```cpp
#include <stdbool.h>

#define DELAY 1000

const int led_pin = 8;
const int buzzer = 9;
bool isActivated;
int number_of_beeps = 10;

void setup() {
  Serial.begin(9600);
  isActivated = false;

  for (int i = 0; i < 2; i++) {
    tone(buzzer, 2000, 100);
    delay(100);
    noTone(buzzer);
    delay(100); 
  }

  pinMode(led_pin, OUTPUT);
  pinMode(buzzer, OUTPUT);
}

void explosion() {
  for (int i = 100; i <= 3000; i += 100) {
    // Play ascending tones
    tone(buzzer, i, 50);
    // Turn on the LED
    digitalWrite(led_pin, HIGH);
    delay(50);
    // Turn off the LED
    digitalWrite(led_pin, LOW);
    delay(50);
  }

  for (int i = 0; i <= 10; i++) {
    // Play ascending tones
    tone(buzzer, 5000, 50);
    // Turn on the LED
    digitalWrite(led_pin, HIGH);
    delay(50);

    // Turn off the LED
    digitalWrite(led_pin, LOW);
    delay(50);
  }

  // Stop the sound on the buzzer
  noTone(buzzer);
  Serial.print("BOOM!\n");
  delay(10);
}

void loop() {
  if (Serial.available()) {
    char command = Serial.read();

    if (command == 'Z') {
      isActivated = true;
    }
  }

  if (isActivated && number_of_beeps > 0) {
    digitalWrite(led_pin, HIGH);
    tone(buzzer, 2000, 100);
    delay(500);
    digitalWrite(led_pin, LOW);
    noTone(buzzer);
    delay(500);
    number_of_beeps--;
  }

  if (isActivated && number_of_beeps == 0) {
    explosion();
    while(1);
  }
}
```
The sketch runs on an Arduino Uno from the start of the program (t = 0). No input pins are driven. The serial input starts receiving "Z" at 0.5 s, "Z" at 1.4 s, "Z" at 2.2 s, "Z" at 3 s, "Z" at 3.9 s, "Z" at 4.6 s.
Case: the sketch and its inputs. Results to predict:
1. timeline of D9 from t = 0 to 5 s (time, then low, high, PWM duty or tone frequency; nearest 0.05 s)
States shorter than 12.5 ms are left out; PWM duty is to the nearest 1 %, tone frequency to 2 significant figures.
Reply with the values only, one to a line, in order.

0 s tone 2000 Hz; 0.1 s low; 0.2 s tone 2000 Hz; 0.3 s low; 0.5 s tone 2000 Hz; 0.6 s low; 1.5 s tone 2000 Hz; 1.6 s low; 2.5 s tone 2000 Hz; 2.6 s low; 3.5 s tone 2000 Hz; 3.6 s low; 4.5 s tone 2000 Hz; 4.6 s low
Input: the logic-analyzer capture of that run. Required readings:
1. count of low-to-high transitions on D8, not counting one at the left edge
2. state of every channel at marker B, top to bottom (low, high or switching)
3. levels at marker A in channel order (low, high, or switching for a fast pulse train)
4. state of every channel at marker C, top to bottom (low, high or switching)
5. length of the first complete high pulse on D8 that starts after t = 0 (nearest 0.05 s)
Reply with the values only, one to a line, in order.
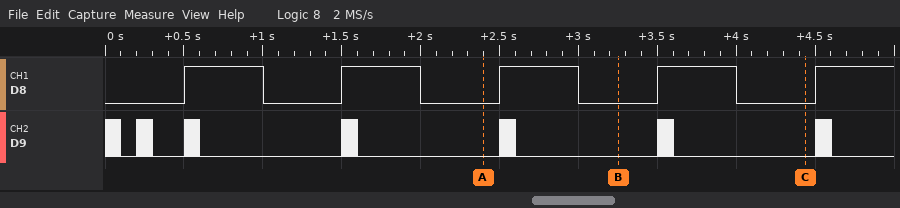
5
D8 low, D9 low
D8 low, D9 low
D8 low, D9 low
0.50 s
